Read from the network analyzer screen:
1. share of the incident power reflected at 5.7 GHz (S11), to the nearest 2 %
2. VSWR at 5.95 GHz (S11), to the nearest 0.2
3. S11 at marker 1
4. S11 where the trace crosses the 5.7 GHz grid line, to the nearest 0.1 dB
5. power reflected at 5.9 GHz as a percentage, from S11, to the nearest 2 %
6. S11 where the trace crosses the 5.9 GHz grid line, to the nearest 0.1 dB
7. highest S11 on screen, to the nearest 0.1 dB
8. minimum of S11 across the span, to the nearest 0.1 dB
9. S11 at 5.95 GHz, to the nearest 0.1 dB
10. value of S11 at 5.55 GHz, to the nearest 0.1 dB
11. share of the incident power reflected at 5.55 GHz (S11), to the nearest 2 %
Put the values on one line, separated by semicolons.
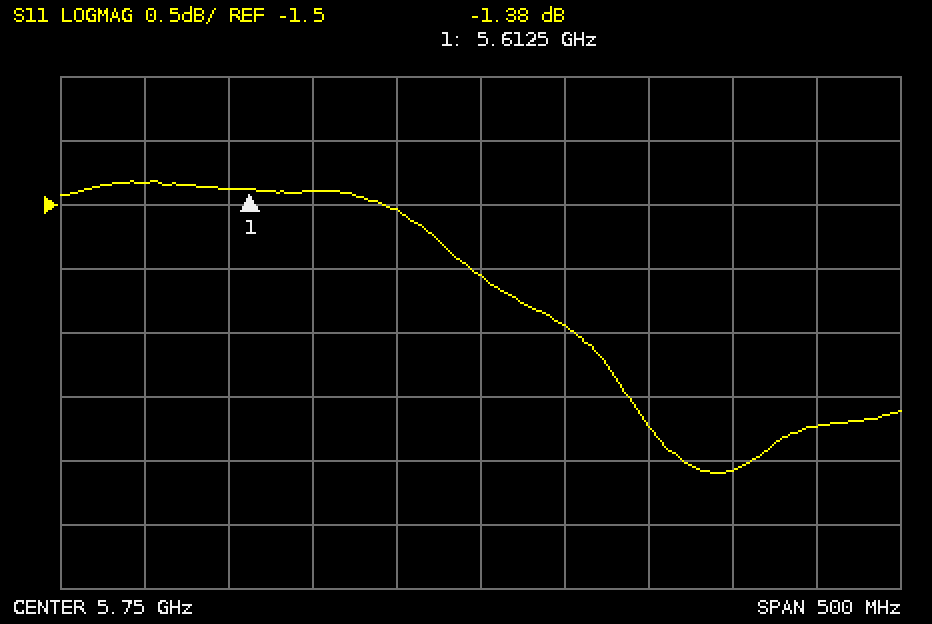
70 %; 5.4; -1.38 dB; -1.5 dB; 44 %; -3.6 dB; -1.3 dB; -3.6 dB; -3.2 dB; -1.3 dB; 74 %
